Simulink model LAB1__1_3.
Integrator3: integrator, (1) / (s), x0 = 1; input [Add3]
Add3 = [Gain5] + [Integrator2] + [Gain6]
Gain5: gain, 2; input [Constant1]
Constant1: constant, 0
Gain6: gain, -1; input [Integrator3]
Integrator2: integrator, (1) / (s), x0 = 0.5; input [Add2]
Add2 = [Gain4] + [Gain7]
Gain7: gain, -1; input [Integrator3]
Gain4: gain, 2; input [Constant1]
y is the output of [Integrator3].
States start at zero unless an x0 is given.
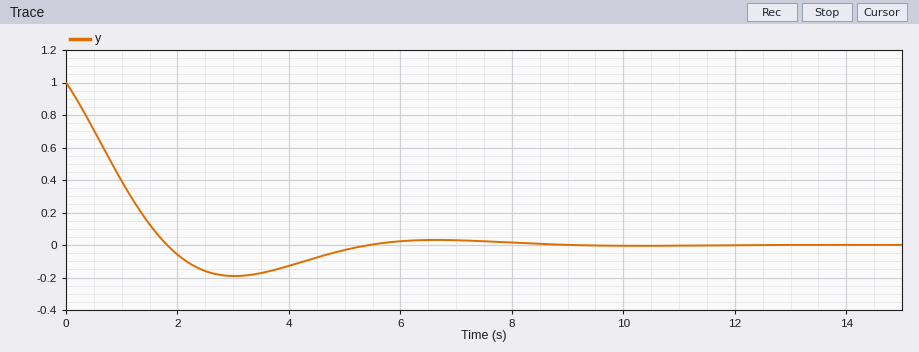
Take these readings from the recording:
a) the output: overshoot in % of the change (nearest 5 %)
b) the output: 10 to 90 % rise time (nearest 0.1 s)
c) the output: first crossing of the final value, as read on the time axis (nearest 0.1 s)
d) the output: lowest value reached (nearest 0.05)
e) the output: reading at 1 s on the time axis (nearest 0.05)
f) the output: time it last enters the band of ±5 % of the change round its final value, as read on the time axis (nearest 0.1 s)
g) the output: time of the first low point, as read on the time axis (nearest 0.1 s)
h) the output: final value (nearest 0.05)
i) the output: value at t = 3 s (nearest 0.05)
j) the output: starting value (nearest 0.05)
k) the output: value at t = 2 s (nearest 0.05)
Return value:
20 %
1.4 s
1.8 s
-0.20
0.40
4.8 s
3.0 s
0.00
-0.20
1.00
-0.05
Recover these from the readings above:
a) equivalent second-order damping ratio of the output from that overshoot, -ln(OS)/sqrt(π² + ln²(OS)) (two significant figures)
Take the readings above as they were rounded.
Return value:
0.46
